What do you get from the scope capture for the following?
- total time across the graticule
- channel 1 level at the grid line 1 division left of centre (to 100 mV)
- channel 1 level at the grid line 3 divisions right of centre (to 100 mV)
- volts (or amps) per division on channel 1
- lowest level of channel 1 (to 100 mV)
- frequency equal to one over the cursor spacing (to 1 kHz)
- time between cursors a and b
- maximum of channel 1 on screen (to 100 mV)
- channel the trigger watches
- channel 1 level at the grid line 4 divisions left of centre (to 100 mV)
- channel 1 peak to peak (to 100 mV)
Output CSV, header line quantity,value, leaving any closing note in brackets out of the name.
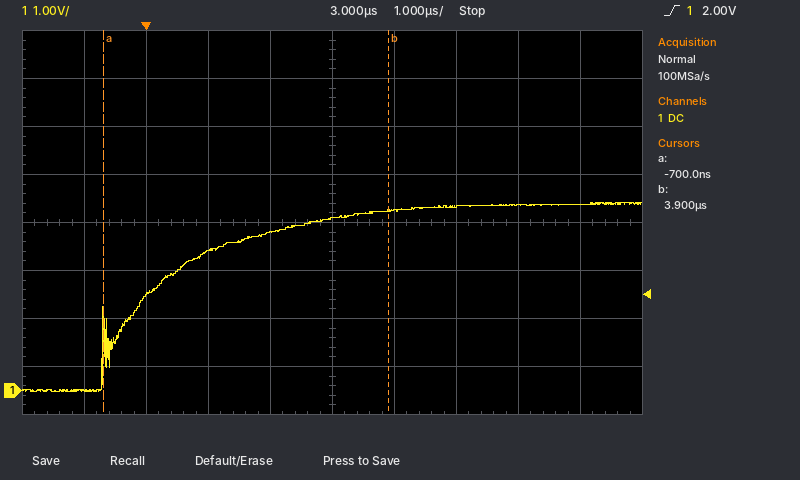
quantity,value
total time across the graticule,10 µs
channel 1 level at the grid line 1 division left of centre,3.3 V
channel 1 level at the grid line 3 divisions right of centre,3.9 V
volts (or amps) per division on channel 1,1 V
lowest level of channel 1,0.0 V
frequency equal to one over the cursor spacing,217 kHz
time between cursors a and b,4.6 µs
maximum of channel 1 on screen,3.9 V
channel the trigger watches,channel 1
channel 1 level at the grid line 4 divisions left of centre,0.0 V
channel 1 peak to peak,3.9 V
